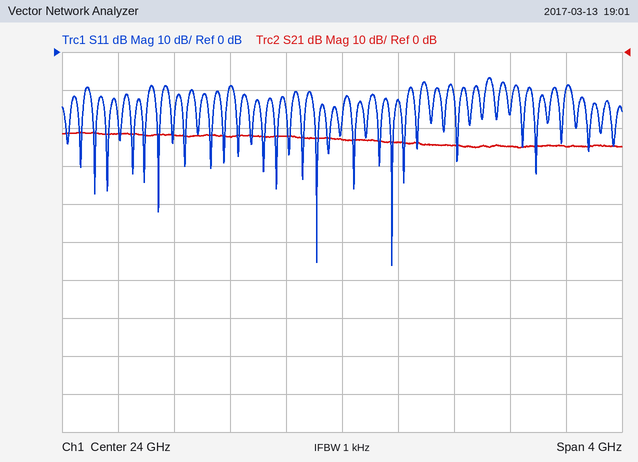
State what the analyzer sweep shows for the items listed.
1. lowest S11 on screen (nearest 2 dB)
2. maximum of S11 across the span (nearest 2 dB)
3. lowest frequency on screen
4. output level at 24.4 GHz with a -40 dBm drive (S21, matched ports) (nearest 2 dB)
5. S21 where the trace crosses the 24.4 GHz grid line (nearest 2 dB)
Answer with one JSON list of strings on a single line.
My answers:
["-56 dB", "-6 dB", "22 GHz", "-64 dBm", "-24 dB"]
